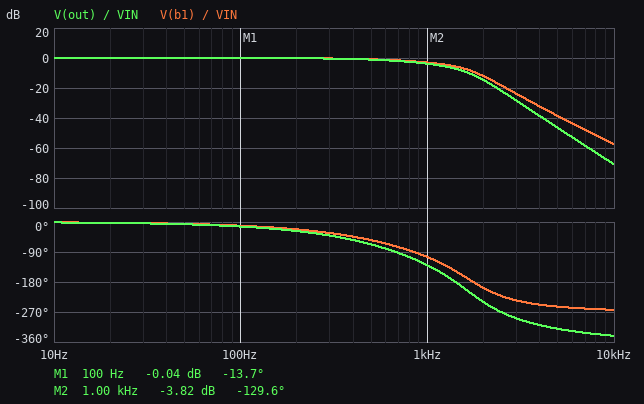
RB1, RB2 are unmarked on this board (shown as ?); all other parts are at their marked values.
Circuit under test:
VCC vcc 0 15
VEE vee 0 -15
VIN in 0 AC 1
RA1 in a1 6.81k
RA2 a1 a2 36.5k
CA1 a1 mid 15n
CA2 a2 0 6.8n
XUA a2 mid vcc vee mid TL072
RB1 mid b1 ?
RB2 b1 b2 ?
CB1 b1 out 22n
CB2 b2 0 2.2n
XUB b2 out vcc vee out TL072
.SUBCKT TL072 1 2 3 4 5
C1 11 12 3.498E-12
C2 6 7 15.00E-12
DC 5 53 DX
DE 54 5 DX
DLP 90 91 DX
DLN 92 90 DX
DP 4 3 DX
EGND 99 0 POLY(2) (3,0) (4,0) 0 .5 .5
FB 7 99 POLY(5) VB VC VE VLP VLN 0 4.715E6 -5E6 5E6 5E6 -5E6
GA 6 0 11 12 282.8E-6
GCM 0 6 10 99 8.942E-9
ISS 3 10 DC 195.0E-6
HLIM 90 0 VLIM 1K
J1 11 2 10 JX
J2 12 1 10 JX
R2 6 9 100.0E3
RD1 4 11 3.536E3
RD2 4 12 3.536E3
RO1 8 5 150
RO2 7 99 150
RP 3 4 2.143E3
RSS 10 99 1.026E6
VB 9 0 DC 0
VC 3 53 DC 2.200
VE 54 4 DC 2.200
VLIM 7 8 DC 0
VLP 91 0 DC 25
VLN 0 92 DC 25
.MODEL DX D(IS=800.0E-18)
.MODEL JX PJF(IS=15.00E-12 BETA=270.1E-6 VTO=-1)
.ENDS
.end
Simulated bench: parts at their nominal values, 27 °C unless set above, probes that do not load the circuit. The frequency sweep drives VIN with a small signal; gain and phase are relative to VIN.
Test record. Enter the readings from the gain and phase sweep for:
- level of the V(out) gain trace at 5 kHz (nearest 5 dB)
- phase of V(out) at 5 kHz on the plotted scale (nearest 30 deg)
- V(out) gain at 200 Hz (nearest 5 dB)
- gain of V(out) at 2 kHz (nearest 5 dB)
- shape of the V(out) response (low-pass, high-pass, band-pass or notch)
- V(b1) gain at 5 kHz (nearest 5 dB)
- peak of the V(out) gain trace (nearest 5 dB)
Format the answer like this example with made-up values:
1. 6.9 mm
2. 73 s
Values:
1. -45 dB
2. -330 deg
3. 0 dB
4. -15 dB
5. low-pass
6. -40 dB
7. 0 dB
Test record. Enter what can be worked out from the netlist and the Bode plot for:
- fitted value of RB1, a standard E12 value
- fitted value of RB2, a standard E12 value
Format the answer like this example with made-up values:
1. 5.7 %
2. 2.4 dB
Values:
1. 5.6 kΩ
2. 33 kΩ
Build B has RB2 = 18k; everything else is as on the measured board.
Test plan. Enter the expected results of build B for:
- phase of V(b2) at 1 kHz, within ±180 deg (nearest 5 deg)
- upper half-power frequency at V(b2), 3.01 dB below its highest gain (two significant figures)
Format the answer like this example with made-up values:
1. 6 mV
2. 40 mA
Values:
1. -110 deg
2. 820 Hz
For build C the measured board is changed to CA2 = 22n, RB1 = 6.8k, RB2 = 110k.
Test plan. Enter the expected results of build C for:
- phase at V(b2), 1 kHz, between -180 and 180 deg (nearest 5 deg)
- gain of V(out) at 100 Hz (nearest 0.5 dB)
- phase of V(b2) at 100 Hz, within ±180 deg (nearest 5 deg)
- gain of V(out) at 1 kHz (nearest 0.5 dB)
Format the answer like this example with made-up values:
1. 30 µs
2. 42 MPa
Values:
1. 145 deg
2. -1.0 dB
3. -40 deg
4. -20.5 dB
